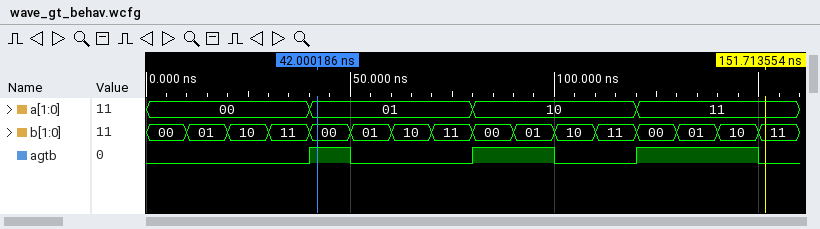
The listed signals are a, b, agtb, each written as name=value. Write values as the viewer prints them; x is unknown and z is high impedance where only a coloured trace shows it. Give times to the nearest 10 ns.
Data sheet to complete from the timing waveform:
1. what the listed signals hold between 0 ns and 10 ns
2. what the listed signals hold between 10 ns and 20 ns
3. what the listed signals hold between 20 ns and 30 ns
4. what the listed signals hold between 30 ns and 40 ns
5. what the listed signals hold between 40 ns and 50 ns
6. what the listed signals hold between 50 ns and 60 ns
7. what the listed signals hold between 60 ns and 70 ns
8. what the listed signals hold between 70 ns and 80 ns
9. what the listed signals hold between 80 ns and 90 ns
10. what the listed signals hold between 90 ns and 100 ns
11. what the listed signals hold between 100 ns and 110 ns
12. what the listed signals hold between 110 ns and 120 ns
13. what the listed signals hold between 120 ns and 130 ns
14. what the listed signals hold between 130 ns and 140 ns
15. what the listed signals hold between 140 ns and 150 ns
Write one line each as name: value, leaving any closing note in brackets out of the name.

what the listed signals hold between 0 ns and 10 ns: a=00, b=00, agtb=0
what the listed signals hold between 10 ns and 20 ns: a=00, b=01, agtb=0
what the listed signals hold between 20 ns and 30 ns: a=00, b=10, agtb=0
what the listed signals hold between 30 ns and 40 ns: a=00, b=11, agtb=0
what the listed signals hold between 40 ns and 50 ns: a=01, b=00, agtb=1
what the listed signals hold between 50 ns and 60 ns: a=01, b=01, agtb=0
what the listed signals hold between 60 ns and 70 ns: a=01, b=10, agtb=0
what the listed signals hold between 70 ns and 80 ns: a=01, b=11, agtb=0
what the listed signals hold between 80 ns and 90 ns: a=10, b=00, agtb=1
what the listed signals hold between 90 ns and 100 ns: a=10, b=01, agtb=1
what the listed signals hold between 100 ns and 110 ns: a=10, b=10, agtb=0
what the listed signals hold between 110 ns and 120 ns: a=10, b=11, agtb=0
what the listed signals hold between 120 ns and 130 ns: a=11, b=00, agtb=1
what the listed signals hold between 130 ns and 140 ns: a=11, b=01, agtb=1
what the listed signals hold between 140 ns and 150 ns: a=11, b=10, agtb=1
